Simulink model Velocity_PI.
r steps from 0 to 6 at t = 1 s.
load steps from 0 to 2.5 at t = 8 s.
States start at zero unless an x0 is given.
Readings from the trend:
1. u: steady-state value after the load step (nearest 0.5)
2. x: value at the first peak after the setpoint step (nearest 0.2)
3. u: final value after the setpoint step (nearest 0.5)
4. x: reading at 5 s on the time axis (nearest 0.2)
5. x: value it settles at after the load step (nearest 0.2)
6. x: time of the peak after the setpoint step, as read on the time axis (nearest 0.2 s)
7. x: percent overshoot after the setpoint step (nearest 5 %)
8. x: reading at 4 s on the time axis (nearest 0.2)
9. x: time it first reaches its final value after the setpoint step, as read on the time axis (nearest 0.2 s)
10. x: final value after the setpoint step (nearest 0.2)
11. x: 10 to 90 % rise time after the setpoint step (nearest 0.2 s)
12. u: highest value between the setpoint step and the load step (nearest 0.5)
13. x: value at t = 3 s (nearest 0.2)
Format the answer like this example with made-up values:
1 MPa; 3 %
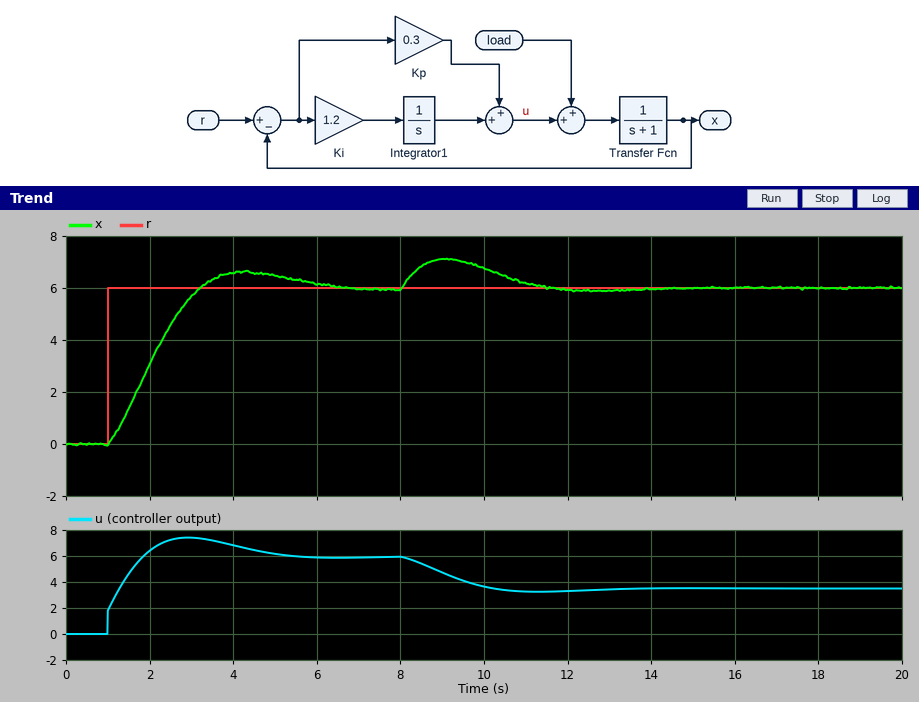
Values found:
3.5; 6.6; 6.0; 6.4; 6.0; 4.2 s; 10 %; 6.6; 3.2 s; 6.0; 1.6 s; 7.5; 5.6
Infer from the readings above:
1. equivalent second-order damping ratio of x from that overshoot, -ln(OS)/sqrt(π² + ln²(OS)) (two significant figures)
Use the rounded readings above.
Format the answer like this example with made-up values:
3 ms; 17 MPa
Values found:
0.59
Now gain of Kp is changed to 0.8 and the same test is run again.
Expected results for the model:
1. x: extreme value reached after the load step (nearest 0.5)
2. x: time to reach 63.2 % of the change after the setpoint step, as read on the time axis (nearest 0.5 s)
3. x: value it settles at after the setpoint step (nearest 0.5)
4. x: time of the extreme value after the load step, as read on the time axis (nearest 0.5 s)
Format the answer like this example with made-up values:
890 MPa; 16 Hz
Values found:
7.0; 2.0 s; 6.0; 9.0 s
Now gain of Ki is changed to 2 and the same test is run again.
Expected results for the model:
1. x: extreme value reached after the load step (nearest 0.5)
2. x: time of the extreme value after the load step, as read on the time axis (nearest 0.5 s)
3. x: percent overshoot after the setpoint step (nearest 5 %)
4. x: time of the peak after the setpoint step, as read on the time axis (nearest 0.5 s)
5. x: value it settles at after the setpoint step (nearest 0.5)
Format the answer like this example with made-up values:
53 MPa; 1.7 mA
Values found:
7.0; 9.0 s; 20 %; 3.5 s; 6.0
